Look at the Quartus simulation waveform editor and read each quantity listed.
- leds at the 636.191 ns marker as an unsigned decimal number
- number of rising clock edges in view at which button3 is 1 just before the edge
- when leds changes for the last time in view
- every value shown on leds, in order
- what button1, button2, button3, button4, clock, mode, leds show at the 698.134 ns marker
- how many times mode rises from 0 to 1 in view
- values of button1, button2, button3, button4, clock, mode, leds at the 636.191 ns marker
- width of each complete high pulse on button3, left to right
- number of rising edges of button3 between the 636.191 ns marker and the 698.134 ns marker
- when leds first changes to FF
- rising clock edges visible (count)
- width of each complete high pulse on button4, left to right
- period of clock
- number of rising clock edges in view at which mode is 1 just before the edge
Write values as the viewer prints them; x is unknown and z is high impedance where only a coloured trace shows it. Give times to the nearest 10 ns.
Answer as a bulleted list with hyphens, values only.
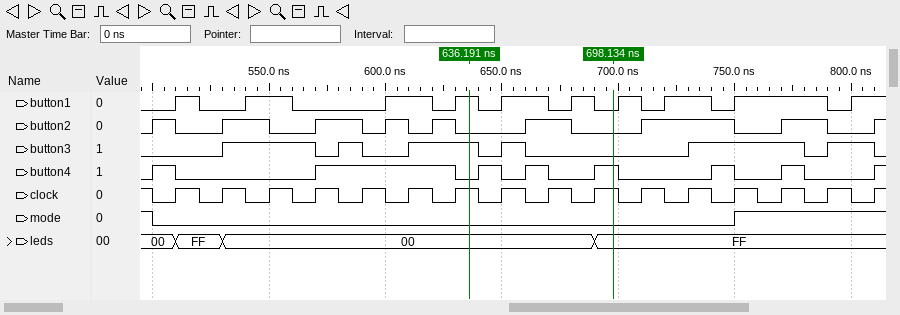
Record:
- 0
- 7
- 690 ns
- 00, FF, 00, FF
- button1=0, button2=0, button3=0, button4=1, clock=1, mode=0, leds=FF
- 1
- button1=1, button2=0, button3=1, button4=0, clock=1, mode=0, leds=00
- 40 ns, 10 ns, 30 ns, 10 ns, 50 ns, 20 ns
- 1
- 510 ns
- 16
- 10 ns, 60 ns, 10 ns, 10 ns, 10 ns, 10 ns, 10 ns
- 20 ns
- 3
